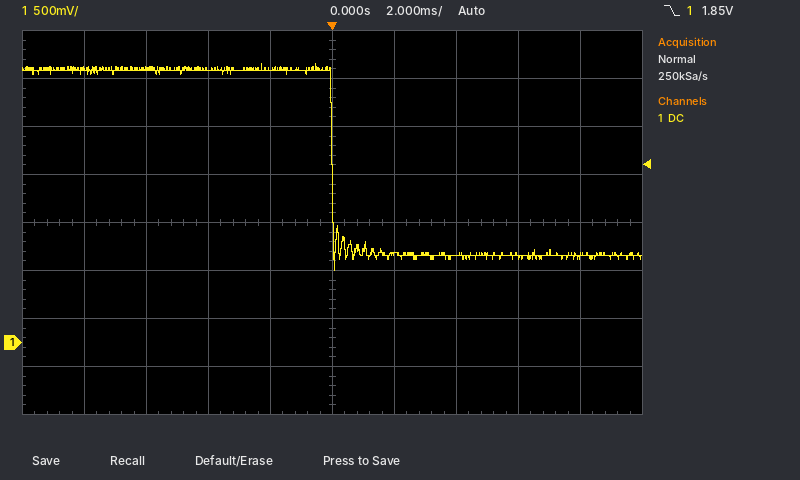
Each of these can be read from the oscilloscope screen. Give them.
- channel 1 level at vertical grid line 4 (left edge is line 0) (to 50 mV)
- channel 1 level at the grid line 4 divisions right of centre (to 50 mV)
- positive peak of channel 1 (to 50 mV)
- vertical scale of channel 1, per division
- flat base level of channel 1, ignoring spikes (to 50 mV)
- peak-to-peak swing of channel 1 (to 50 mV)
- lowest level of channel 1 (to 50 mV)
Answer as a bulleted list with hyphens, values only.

- 2.85 V
- 900 mV
- 2.90 V
- 500 mV
- 900 mV
- 2.15 V
- 750 mV
